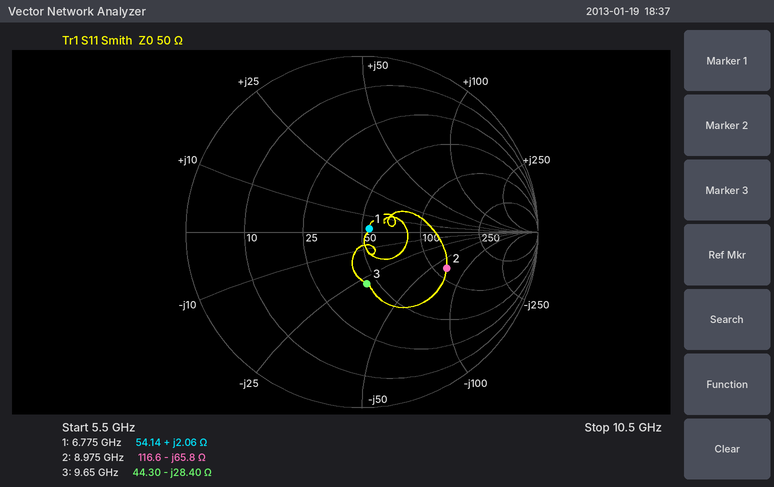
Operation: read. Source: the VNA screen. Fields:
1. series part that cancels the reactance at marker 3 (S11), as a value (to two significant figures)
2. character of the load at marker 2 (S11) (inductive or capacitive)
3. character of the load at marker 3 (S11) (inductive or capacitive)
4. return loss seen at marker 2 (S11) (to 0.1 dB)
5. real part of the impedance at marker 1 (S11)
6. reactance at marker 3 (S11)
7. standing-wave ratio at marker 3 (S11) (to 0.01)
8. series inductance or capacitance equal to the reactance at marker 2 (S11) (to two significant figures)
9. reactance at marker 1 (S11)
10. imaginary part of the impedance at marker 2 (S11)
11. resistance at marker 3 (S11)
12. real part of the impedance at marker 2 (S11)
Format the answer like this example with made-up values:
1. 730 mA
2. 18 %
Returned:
1. 470 pH
2. capacitive
3. capacitive
4. 5.6 dB
5. 54.14 Ω
6. -28.40 Ω
7. 1.83
8. 270 fF
9. +2.06 Ω
10. -65.8 Ω
11. 44.30 Ω
12. 116.6 Ω
